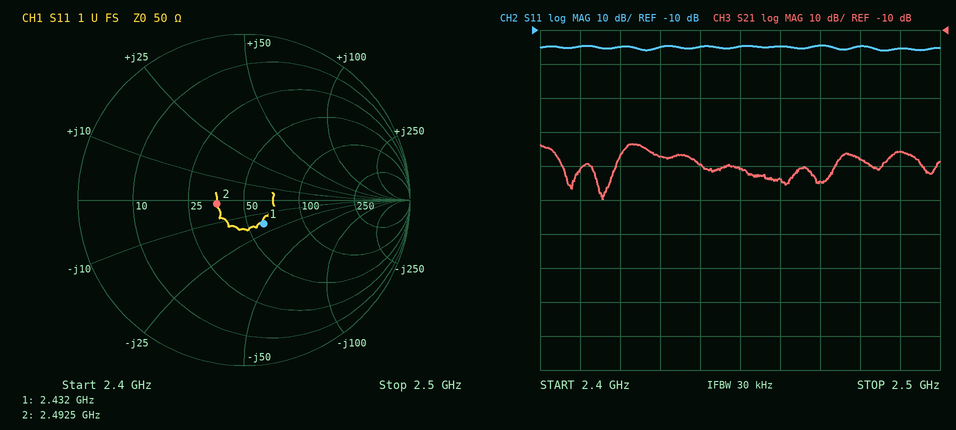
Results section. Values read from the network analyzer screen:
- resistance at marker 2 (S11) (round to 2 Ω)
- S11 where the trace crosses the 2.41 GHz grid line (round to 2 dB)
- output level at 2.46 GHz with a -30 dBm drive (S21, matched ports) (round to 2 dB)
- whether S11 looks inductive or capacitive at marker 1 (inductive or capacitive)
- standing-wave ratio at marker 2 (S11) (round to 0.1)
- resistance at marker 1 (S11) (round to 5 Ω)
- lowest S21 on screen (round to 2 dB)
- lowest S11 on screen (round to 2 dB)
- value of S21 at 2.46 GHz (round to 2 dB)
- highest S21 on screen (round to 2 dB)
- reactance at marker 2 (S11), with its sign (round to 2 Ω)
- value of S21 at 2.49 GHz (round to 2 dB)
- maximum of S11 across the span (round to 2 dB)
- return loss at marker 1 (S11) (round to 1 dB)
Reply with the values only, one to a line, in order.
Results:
36 Ω
-14 dB
-84 dBm
capacitive
1.4
60 Ω
-60 dB
-16 dB
-54 dB
-44 dB
-2 Ω
-46 dB
-14 dB
15 dB
